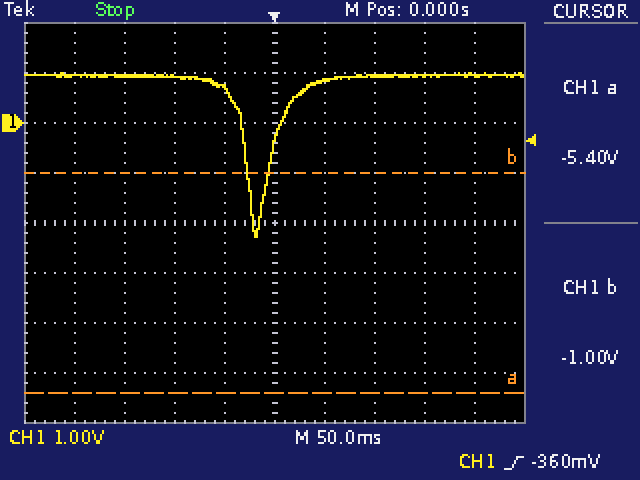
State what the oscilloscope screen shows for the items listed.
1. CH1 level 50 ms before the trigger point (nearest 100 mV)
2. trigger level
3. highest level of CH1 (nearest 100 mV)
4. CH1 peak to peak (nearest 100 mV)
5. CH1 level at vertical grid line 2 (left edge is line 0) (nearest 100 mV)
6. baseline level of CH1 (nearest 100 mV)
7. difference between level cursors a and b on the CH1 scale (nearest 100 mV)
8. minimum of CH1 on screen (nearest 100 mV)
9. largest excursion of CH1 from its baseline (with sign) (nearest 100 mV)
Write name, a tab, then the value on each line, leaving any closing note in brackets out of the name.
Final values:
CH1 level 50 ms before the trigger point	700 mV
trigger level	-360 mV
highest level of CH1	1.0 V
CH1 peak to peak	3.3 V
CH1 level at vertical grid line 2 (left edge is line 0)	900 mV
baseline level of CH1	900 mV
difference between level cursors a and b on the CH1 scale	4.4 V
minimum of CH1 on screen	-2.3 V
largest excursion of CH1 from its baseline (with sign)	-3.2 V
